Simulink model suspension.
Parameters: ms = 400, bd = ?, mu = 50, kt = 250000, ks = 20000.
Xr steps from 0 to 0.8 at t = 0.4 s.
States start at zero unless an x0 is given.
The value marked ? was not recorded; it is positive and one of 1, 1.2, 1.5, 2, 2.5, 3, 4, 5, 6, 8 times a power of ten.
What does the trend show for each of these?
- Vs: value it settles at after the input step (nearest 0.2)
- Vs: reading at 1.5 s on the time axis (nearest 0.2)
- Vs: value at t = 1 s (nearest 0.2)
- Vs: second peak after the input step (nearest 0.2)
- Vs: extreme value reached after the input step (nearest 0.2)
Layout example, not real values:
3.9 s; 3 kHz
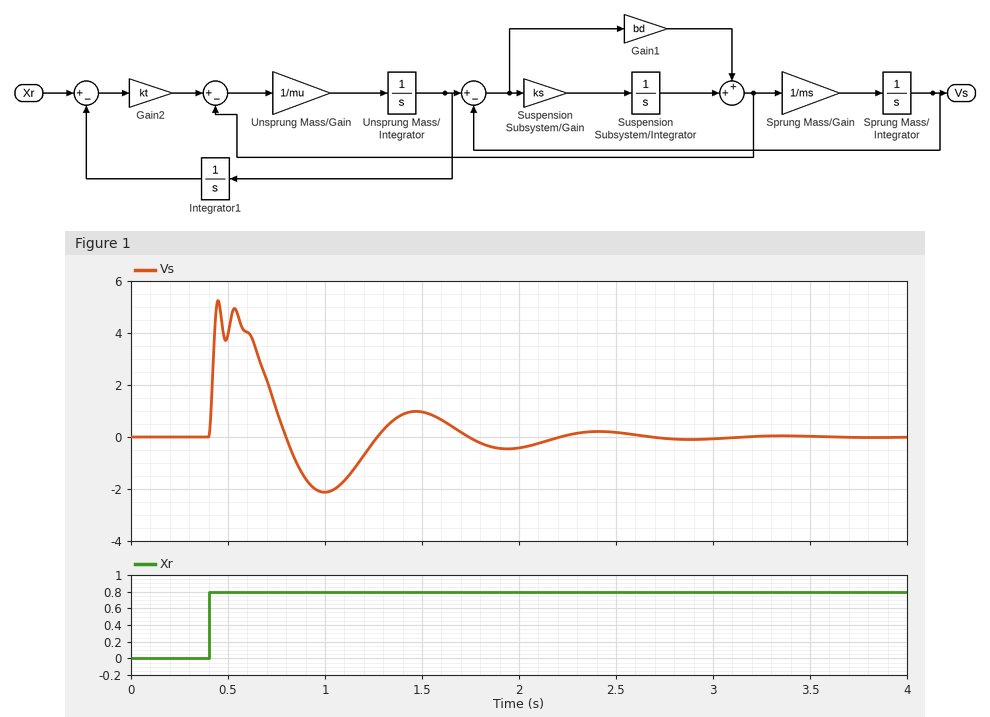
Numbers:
0.0; 1.0; -2.2; 5.0; 5.2
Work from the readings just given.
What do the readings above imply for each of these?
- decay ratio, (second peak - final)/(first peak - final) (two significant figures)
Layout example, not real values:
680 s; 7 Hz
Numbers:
0.96
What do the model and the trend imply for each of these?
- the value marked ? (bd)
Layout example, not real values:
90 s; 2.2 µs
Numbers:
1500
